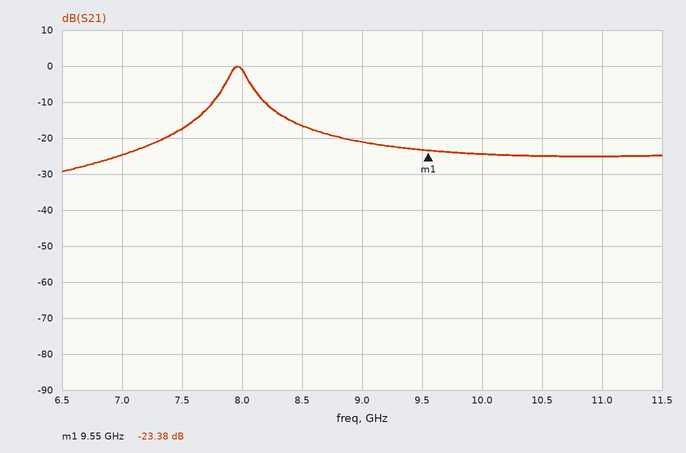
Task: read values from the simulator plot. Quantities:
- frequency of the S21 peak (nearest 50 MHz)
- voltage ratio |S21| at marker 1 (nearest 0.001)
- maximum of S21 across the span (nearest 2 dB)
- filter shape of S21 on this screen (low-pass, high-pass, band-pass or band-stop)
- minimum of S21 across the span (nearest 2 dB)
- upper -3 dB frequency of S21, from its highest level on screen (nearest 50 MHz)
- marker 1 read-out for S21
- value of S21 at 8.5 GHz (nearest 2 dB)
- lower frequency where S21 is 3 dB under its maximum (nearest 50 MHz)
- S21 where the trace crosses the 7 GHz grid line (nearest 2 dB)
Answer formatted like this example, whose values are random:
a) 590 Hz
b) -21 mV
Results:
a) 7.95 GHz
b) 0.068
c) 0 dB
d) band-pass
e) -30 dB
f) 8.05 GHz
g) -23.38 dB
h) -16 dB
i) 7.90 GHz
j) -24 dB
